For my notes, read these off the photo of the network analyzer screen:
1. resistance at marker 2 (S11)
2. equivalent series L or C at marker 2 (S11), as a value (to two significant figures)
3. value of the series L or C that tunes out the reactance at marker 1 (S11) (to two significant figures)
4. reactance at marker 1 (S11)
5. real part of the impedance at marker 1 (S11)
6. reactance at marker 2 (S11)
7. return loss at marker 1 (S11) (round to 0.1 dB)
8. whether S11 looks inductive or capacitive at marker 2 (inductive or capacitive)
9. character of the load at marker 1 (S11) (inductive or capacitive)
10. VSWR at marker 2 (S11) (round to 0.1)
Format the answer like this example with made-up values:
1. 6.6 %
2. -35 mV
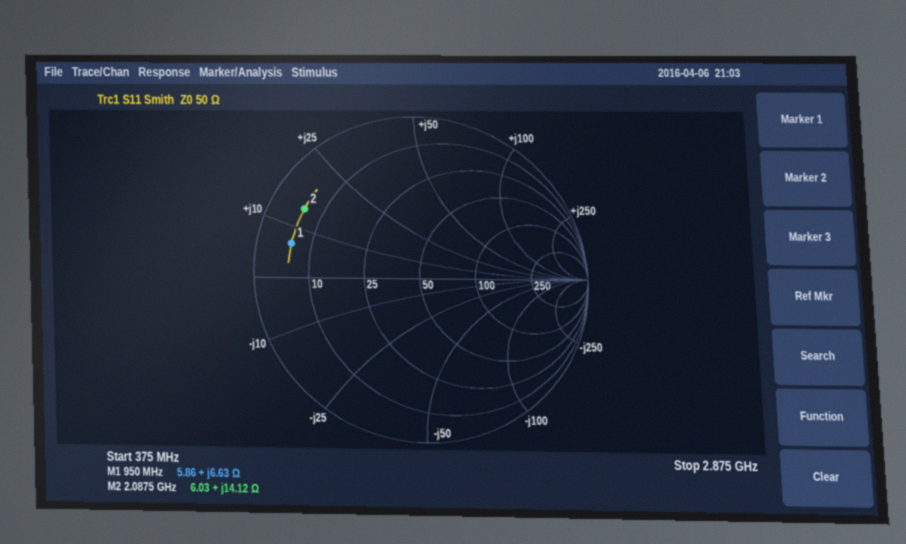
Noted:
1. 6.03 Ω
2. 1.1 nH
3. 25 pF
4. +6.63 Ω
5. 5.86 Ω
6. +14.12 Ω
7. 2.0 dB
8. inductive
9. inductive
10. 9.0
